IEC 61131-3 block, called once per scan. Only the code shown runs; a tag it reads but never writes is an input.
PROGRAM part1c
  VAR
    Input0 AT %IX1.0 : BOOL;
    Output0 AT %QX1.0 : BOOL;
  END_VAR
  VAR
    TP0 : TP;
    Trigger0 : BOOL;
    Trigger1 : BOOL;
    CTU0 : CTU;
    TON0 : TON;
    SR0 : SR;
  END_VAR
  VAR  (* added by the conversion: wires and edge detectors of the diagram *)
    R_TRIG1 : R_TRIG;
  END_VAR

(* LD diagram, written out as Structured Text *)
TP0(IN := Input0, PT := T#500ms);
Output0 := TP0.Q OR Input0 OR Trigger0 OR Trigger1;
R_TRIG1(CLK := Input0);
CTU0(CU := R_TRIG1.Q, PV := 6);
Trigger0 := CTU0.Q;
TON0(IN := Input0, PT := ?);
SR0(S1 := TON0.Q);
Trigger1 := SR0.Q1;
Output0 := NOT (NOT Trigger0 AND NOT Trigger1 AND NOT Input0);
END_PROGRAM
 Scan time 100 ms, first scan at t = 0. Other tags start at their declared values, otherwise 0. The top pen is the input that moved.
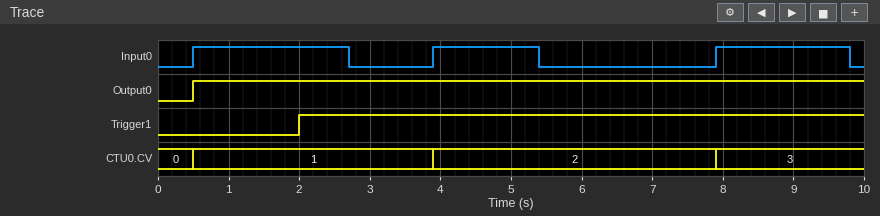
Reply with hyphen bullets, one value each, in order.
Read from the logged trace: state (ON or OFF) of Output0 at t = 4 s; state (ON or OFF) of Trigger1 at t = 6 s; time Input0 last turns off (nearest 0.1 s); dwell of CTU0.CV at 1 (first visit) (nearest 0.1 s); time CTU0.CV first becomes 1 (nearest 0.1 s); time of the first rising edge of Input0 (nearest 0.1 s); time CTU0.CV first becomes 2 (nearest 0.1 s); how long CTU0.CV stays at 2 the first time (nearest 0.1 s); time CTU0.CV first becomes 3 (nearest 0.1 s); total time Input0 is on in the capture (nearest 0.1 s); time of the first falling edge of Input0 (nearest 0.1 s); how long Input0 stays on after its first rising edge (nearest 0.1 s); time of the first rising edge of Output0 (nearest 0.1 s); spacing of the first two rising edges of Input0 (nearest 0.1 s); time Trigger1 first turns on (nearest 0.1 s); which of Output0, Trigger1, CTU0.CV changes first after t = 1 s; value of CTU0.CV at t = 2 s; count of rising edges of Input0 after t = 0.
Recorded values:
- ON
- ON
- 9.8 s
- 3.4 s
- 0.5 s
- 0.5 s
- 3.9 s
- 4.0 s
- 7.9 s
- 5.6 s
- 2.7 s
- 2.2 s
- 0.5 s
- 3.4 s
- 2.0 s
- Trigger1
- 1
- 3
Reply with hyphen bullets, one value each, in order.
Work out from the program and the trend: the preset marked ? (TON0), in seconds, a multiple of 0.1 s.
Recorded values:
- 1.5 s
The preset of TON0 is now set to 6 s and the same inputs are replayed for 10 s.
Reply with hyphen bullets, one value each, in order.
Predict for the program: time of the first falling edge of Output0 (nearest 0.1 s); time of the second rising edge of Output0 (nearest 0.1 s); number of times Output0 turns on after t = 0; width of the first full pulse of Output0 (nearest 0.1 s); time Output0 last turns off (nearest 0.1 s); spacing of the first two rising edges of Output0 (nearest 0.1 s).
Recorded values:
- 2.7 s
- 3.9 s
- 3
- 2.2 s
- 9.8 s
- 3.4 s
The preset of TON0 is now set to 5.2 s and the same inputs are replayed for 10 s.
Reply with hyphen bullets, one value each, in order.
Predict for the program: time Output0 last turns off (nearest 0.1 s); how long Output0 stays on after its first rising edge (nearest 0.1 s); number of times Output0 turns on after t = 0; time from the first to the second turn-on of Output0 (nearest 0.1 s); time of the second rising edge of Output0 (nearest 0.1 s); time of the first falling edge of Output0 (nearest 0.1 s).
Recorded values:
- 9.8 s
- 2.2 s
- 3
- 3.4 s
- 3.9 s
- 2.7 s
